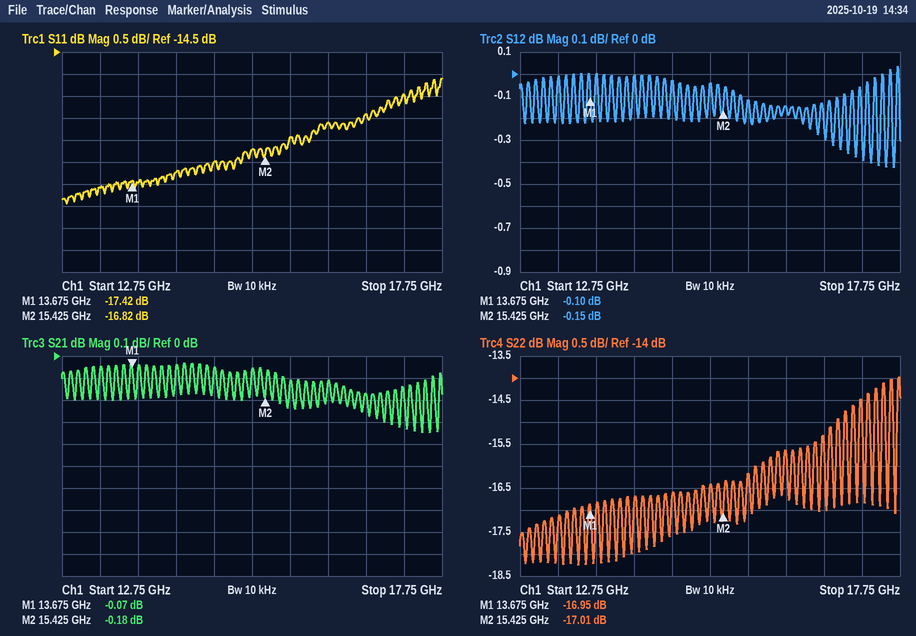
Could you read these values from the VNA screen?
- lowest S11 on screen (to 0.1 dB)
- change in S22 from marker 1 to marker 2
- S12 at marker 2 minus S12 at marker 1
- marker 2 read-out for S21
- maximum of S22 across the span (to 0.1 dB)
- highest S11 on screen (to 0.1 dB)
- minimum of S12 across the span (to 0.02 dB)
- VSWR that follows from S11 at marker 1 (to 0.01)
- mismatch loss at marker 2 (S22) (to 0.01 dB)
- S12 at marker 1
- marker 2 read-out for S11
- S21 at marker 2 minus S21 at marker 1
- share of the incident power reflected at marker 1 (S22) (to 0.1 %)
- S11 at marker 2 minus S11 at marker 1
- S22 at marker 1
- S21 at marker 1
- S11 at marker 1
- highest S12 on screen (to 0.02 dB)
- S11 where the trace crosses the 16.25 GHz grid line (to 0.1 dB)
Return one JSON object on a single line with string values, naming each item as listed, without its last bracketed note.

{"lowest S11 on screen": "-17.9 dB", "change in S22 from marker 1 to marker 2": "-0.06 dB", "S12 at marker 2 minus S12 at marker 1": "-0.05 dB", "marker 2 read-out for S21": "-0.18 dB", "maximum of S22 across the span": "-14.0 dB", "highest S11 on screen": "-15.1 dB", "minimum of S12 across the span": "-0.42 dB", "VSWR that follows from S11 at marker 1": "1.31", "mismatch loss at marker 2 (S22)": "0.09 dB", "S12 at marker 1": "-0.10 dB", "marker 2 read-out for S11": "-16.82 dB", "S21 at marker 2 minus S21 at marker 1": "-0.11 dB", "share of the incident power reflected at marker 1 (S22)": "2.0 %", "S11 at marker 2 minus S11 at marker 1": "0.60 dB", "S22 at marker 1": "-16.95 dB", "S21 at marker 1": "-0.07 dB", "S11 at marker 1": "-17.42 dB", "highest S12 on screen": "0.04 dB", "S11 where the trace crosses the 16.25 GHz grid line": "-16.1 dB"}
